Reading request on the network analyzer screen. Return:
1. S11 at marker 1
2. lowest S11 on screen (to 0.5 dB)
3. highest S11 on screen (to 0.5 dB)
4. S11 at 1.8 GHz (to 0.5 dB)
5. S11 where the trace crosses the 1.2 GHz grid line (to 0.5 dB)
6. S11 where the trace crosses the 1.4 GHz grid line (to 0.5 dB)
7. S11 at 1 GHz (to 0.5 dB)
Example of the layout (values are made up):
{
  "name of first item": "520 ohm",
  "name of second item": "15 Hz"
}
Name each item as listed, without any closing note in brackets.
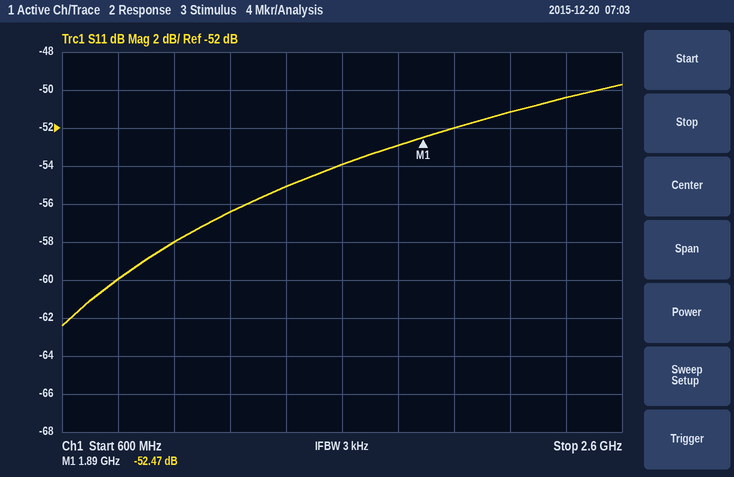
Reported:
{
  "S11 at marker 1": "-52.47 dB",
  "lowest S11 on screen": "-62.5 dB",
  "highest S11 on screen": "-49.5 dB",
  "S11 at 1.8 GHz": "-53.0 dB",
  "S11 where the trace crosses the 1.2 GHz grid line": "-56.5 dB",
  "S11 where the trace crosses the 1.4 GHz grid line": "-55.0 dB",
  "S11 at 1 GHz": "-58.0 dB"
}
